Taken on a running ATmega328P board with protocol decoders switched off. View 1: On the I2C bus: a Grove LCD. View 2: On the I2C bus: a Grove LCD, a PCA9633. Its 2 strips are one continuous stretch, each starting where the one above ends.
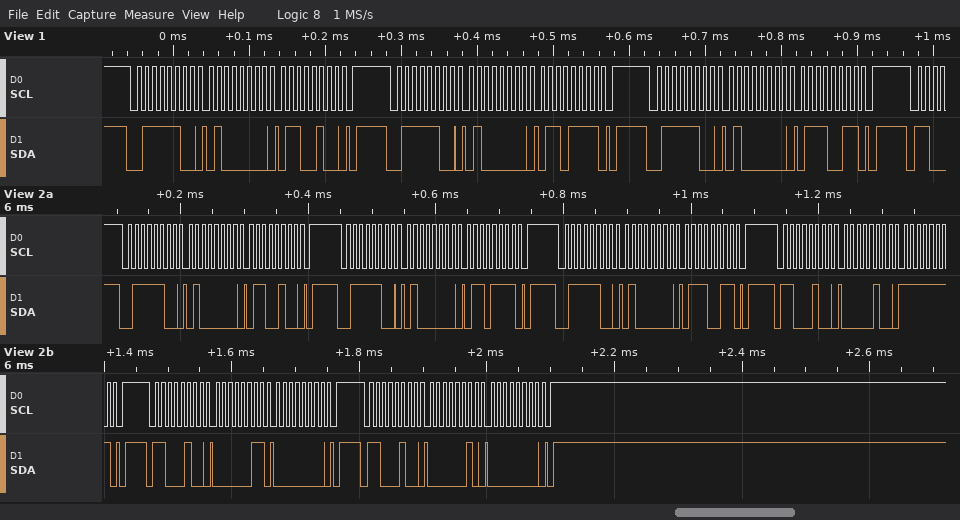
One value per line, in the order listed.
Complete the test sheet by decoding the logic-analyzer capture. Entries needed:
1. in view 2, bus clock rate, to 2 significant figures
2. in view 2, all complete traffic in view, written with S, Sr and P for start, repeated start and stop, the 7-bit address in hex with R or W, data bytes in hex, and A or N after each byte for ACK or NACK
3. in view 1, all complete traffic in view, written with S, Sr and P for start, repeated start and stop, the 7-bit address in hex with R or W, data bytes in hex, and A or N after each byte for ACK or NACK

100 kHz
S 3EW A 40 A 64 A P S 3EW A 40 A 6F A P S 3EW A 40 A 73 A P S 62W A 04 A FF A P S 62W A 03 A 00 A P S 62W A 02 A 00 A P
S 3EW A 40 A 64 A P S 3EW A 40 A 6F A P S 3EW A 40 A 73 A P
